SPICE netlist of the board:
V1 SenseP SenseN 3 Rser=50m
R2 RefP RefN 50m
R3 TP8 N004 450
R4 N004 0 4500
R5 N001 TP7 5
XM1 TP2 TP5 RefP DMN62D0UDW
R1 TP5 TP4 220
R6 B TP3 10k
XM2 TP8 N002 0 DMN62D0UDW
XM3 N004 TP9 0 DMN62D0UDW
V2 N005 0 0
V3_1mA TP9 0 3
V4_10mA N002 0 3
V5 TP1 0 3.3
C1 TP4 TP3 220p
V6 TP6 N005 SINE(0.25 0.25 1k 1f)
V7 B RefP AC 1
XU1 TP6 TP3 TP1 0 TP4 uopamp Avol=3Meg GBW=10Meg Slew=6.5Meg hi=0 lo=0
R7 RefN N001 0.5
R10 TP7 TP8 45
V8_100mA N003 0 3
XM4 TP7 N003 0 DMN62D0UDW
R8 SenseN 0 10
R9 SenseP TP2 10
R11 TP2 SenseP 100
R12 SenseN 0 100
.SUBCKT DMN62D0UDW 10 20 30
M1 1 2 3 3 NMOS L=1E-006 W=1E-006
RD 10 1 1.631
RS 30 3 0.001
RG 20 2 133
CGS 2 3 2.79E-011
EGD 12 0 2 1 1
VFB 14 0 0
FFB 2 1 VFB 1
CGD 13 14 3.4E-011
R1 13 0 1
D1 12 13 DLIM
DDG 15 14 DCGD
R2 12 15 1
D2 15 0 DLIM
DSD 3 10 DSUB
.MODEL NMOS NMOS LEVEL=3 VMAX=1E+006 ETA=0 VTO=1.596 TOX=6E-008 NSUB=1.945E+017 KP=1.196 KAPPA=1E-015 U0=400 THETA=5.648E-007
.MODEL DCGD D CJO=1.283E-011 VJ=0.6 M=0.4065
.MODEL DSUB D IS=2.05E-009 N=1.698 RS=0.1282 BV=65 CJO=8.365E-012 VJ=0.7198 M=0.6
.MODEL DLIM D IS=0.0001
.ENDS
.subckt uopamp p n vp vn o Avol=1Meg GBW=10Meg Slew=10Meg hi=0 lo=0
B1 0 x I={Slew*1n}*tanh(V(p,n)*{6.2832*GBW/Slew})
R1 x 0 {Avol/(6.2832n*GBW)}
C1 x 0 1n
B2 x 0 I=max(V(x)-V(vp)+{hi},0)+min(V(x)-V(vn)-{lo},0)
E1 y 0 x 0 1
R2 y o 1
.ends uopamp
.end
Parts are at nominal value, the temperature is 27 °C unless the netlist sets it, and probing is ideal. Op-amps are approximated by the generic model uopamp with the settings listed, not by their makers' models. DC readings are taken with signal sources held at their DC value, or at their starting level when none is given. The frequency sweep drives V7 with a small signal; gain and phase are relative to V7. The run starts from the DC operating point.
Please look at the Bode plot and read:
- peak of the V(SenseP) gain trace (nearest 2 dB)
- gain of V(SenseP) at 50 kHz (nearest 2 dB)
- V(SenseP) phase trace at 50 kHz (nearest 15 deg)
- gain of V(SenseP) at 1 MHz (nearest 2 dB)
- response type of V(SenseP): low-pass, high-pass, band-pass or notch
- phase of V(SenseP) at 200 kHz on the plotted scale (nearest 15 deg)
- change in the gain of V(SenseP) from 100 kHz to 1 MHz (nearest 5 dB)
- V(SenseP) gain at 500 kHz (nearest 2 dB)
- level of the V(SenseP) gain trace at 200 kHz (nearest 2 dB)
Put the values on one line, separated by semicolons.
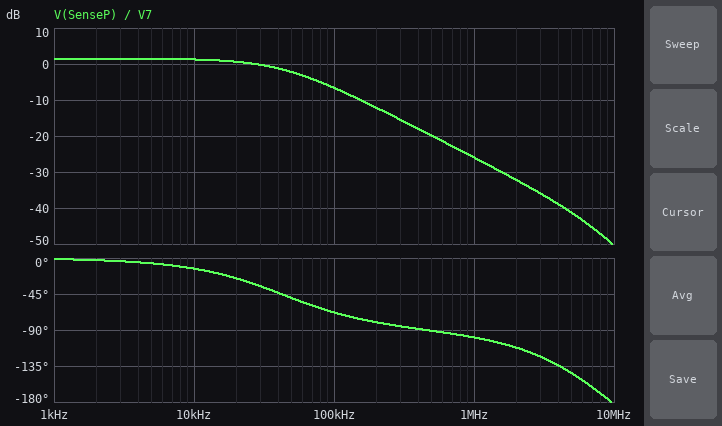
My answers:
2 dB; -2 dB; -45 deg; -26 dB; low-pass; -75 deg; -20 dB; -20 dB; -12 dB
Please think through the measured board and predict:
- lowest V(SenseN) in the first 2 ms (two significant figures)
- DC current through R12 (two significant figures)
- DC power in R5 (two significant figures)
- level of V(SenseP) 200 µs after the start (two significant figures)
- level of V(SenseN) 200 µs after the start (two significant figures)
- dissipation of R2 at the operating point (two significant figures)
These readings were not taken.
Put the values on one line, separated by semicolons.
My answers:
-590 mV; 3.0 mA; 5.3 mW; 2.4 V; -580 mV; 53 µW
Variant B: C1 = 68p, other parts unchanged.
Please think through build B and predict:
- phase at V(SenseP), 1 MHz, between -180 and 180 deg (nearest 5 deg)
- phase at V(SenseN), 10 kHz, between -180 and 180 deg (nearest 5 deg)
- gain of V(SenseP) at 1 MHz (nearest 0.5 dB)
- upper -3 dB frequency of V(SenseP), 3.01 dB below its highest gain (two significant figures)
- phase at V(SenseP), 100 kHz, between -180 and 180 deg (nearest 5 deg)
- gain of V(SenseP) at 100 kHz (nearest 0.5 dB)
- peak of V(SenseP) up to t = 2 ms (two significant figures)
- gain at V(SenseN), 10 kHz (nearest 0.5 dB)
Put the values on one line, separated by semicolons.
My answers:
-95 deg; -5 deg; -16.0 dB; 140 kHz; -35 deg; -0.5 dB; 3.0 V; 1.5 dB
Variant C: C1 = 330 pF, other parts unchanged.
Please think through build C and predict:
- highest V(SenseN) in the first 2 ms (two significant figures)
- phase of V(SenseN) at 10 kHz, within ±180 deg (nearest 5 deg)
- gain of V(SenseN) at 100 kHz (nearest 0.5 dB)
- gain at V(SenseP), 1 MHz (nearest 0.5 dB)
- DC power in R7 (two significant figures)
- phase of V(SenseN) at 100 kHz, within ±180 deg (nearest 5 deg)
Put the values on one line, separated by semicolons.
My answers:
-2.1 mV; -20 deg; -10.0 dB; -29.5 dB; 530 µW; -75 deg
